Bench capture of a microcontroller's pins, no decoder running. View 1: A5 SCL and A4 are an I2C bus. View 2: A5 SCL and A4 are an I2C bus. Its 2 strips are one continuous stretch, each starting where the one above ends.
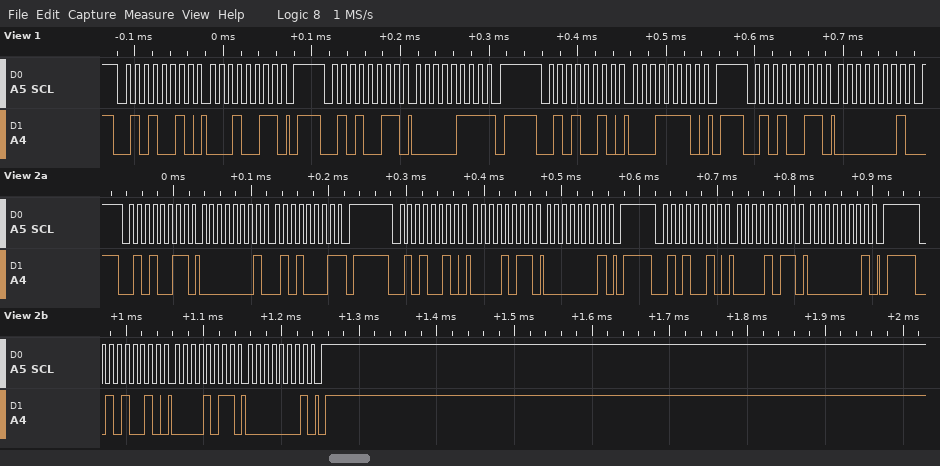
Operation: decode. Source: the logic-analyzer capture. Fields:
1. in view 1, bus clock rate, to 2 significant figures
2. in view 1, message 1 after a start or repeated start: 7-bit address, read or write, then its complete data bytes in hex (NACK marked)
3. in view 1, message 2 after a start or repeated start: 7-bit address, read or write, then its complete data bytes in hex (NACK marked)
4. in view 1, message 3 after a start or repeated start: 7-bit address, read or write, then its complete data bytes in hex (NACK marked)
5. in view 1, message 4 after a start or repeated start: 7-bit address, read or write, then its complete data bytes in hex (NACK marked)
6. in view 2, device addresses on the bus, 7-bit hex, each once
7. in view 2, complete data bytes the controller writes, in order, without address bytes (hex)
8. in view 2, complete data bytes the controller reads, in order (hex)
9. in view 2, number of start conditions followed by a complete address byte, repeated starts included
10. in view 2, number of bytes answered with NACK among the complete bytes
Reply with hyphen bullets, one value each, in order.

- 100 kHz
- 0x29 write: 13
- 0x29 read: 07 NACK
- 0x29 write: 1E
- 0x29 read: 01
- 0x29
- 0B 01 0B 01 0B 01
- 01 51
- 4
- 1
